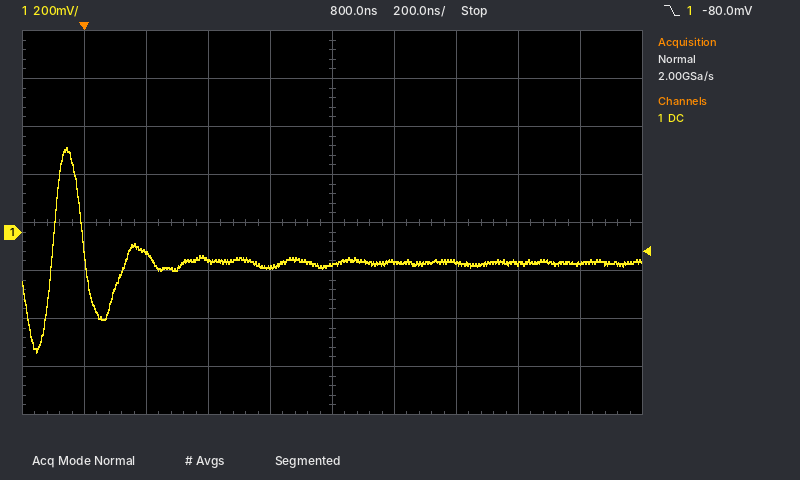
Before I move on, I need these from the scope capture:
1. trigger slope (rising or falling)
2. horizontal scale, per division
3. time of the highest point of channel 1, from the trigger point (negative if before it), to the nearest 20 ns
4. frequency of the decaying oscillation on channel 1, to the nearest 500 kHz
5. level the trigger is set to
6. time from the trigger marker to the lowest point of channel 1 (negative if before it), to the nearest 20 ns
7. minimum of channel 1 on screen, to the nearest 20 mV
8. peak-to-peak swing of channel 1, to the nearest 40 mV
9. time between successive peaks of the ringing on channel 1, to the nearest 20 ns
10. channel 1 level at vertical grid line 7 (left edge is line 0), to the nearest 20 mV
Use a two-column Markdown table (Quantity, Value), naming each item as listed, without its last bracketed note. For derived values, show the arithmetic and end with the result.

| Quantity | Value |
|---|---|
| trigger slope | falling |
| horizontal scale, per division | 200 ns |
| time of the highest point of channel 1, from the trigger point (negative if before it), to the nearest 20 ns | -60 ns |
| frequency of the decaying oscillation on channel 1, to the nearest 500 kHz | 1 / 220 ns ≈ 4.5 MHz |
| level the trigger is set to | -80.0 mV |
| time from the trigger marker to the lowest point of channel 1 (negative if before it), to the nearest 20 ns | -160 ns |
| minimum of channel 1 on screen, to the nearest 20 mV | -500 mV |
| peak-to-peak swing of channel 1, to the nearest 40 mV | 840 mV |
| time between successive peaks of the ringing on channel 1, to the nearest 20 ns | 220 ns |
| channel 1 level at vertical grid line 7 (left edge is line 0), to the nearest 20 mV | -120 mV |
